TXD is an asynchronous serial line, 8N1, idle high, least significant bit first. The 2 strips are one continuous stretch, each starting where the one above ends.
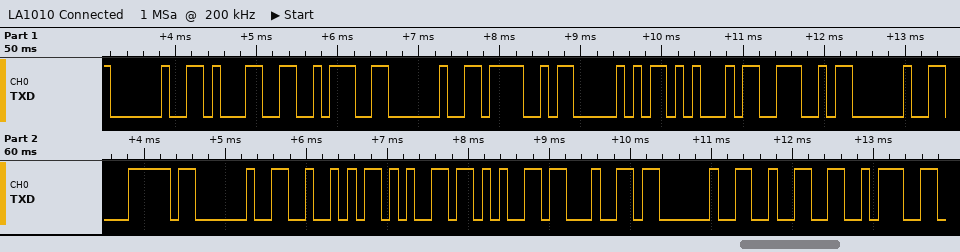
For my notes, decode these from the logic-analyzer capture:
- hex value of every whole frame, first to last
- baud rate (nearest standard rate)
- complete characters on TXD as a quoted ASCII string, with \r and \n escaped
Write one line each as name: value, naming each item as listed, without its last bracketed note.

hex value of every whole frame, first to last: 20 31 3A 20 4F 50 45 4E 20 7C 20 52 65 65 64 20 32 3A
baud rate: 9600 baud
complete characters on TXD as a quoted ASCII string, with \r and \n escaped: " 1: OPEN | Reed 2:"
